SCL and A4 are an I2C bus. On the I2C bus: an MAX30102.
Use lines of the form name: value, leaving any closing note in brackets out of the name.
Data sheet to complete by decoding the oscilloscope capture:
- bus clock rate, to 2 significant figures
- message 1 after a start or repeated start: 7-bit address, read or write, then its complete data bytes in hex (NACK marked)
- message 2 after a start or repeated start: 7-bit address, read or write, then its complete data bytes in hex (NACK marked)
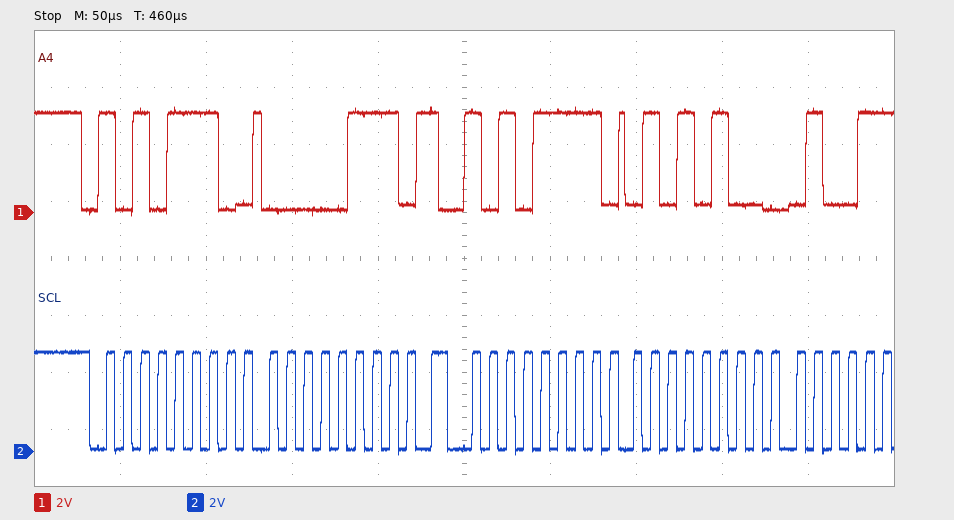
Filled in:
bus clock rate, to 2 significant figures: 100 kHz
message 1 after a start or repeated start: 7-bit address, read or write, then its complete data bytes in hex: 0x57 write: 07
message 2 after a start or repeated start: 7-bit address, read or write, then its complete data bytes in hex: 0x57 read: 54
